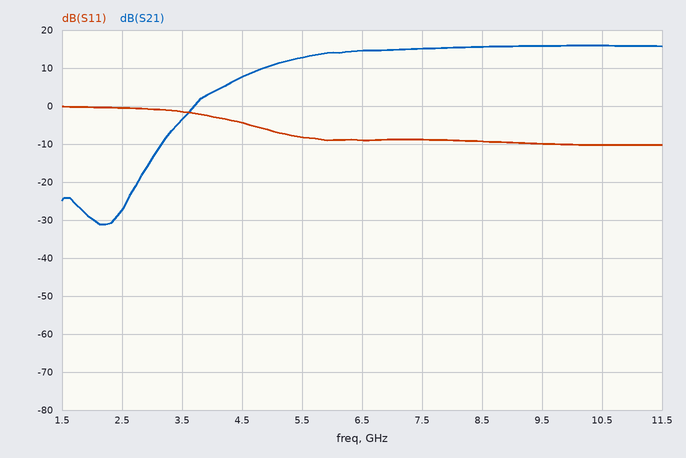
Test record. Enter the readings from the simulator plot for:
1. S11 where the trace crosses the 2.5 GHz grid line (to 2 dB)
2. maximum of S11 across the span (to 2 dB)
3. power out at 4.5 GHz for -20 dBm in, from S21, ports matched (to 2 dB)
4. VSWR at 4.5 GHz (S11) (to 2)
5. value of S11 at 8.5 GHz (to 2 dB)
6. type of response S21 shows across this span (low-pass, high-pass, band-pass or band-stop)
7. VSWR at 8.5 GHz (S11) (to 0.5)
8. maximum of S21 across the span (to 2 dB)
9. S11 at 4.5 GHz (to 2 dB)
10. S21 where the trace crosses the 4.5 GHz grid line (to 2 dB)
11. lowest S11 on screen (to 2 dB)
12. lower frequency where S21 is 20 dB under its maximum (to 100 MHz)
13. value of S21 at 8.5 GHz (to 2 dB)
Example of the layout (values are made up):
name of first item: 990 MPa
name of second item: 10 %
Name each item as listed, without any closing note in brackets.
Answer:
S11 where the trace crosses the 2.5 GHz grid line: 0 dB
maximum of S11 across the span: 0 dB
power out at 4.5 GHz for -20 dBm in, from S21, ports matched: -12 dBm
VSWR at 4.5 GHz (S11): 4
value of S11 at 8.5 GHz: -10 dB
type of response S21 shows across this span: high-pass
VSWR at 8.5 GHz (S11): 2.0
maximum of S21 across the span: 16 dB
S11 at 4.5 GHz: -4 dB
S21 where the trace crosses the 4.5 GHz grid line: 8 dB
lowest S11 on screen: -10 dB
lower frequency where S21 is 20 dB under its maximum: 3.5 GHz
value of S21 at 8.5 GHz: 16 dB
